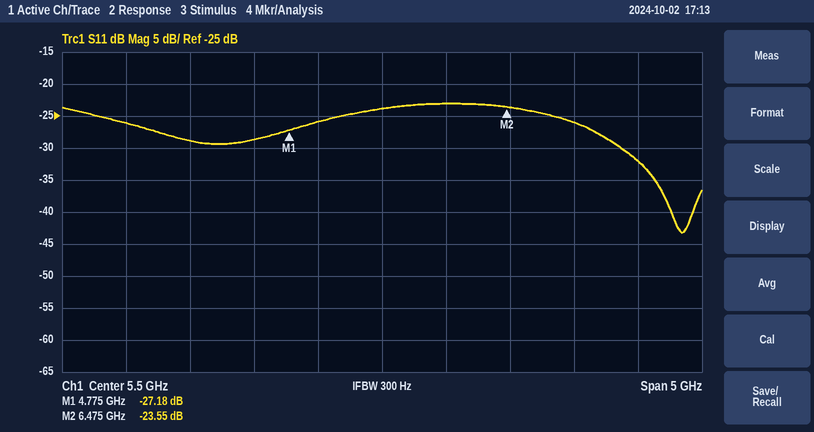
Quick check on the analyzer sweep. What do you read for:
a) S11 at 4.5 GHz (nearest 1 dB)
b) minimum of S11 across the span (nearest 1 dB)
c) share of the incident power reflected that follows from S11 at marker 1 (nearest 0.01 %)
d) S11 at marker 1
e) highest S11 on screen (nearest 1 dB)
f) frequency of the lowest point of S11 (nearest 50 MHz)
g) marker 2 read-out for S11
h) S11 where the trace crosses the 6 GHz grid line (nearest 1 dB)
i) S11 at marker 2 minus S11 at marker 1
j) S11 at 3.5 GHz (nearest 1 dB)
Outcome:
-29 dB
-43 dB
0.19 %
-27.18 dB
-23 dB
7.85 GHz
-23.55 dB
-23 dB
3.63 dB
-26 dB
